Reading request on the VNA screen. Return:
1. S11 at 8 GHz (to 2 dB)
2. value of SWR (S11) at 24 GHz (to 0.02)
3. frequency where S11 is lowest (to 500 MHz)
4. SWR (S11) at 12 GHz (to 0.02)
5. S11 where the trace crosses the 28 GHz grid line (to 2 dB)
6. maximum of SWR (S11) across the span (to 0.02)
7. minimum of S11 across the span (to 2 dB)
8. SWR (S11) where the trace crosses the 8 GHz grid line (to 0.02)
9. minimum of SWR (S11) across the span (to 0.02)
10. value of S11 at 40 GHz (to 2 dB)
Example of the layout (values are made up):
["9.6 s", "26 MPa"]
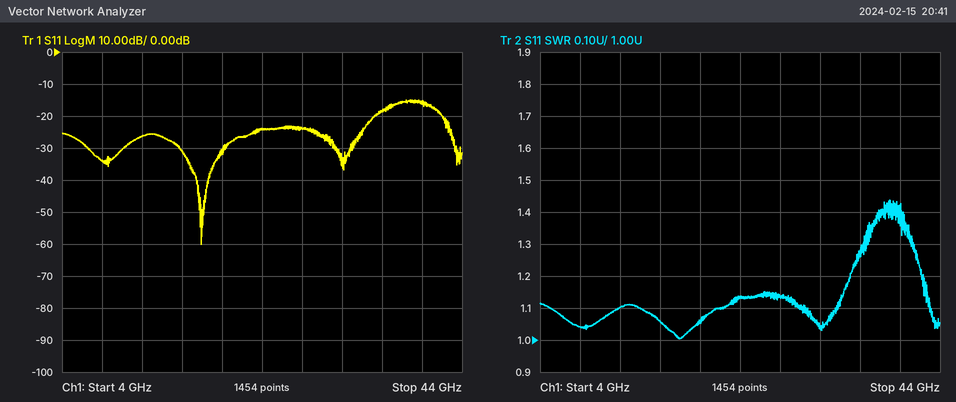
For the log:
["-34 dB", "1.14", "18.0 GHz", "1.10", "-24 dB", "1.44", "-60 dB", "1.04", "1.00", "-16 dB"]
